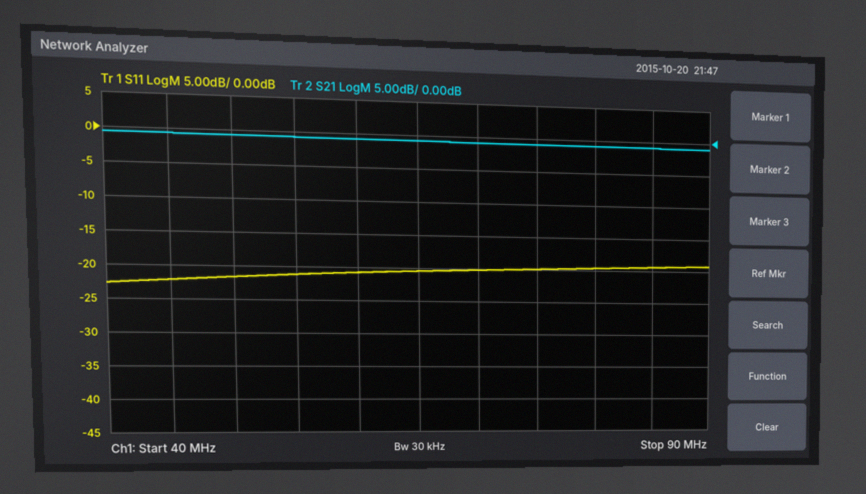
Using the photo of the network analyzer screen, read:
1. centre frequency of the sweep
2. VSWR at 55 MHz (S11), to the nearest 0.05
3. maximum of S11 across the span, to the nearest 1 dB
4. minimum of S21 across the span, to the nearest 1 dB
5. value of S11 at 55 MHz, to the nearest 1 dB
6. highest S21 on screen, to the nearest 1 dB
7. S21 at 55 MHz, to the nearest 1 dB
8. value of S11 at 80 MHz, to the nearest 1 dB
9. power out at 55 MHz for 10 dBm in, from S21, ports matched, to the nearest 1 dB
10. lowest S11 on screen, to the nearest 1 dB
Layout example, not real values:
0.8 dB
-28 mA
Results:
65 MHz
1.20
-19 dB
-1 dB
-21 dB
-1 dB
-1 dB
-20 dB
9 dBm
-23 dB
